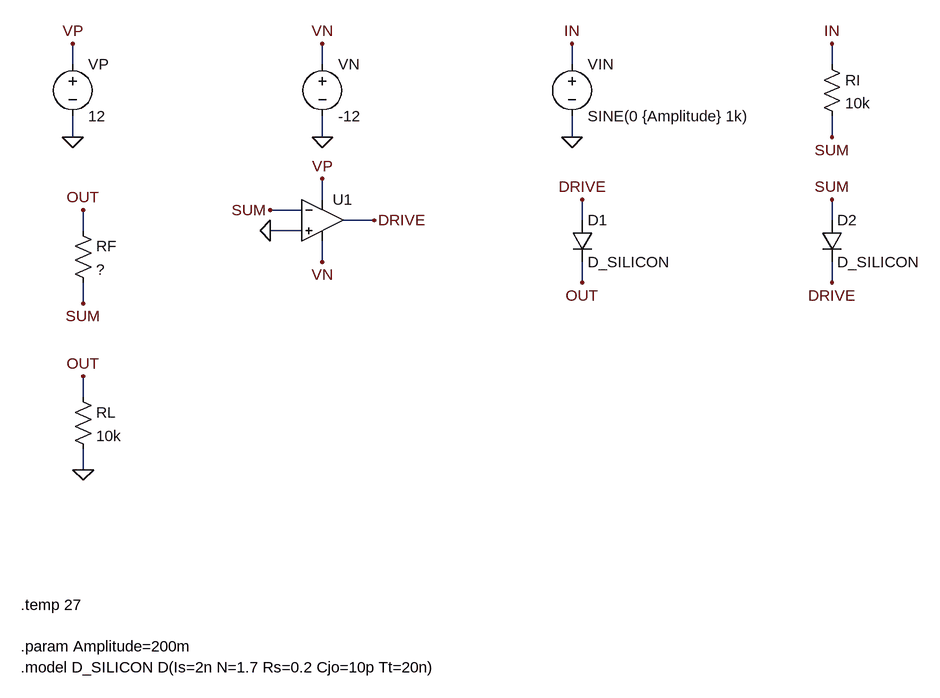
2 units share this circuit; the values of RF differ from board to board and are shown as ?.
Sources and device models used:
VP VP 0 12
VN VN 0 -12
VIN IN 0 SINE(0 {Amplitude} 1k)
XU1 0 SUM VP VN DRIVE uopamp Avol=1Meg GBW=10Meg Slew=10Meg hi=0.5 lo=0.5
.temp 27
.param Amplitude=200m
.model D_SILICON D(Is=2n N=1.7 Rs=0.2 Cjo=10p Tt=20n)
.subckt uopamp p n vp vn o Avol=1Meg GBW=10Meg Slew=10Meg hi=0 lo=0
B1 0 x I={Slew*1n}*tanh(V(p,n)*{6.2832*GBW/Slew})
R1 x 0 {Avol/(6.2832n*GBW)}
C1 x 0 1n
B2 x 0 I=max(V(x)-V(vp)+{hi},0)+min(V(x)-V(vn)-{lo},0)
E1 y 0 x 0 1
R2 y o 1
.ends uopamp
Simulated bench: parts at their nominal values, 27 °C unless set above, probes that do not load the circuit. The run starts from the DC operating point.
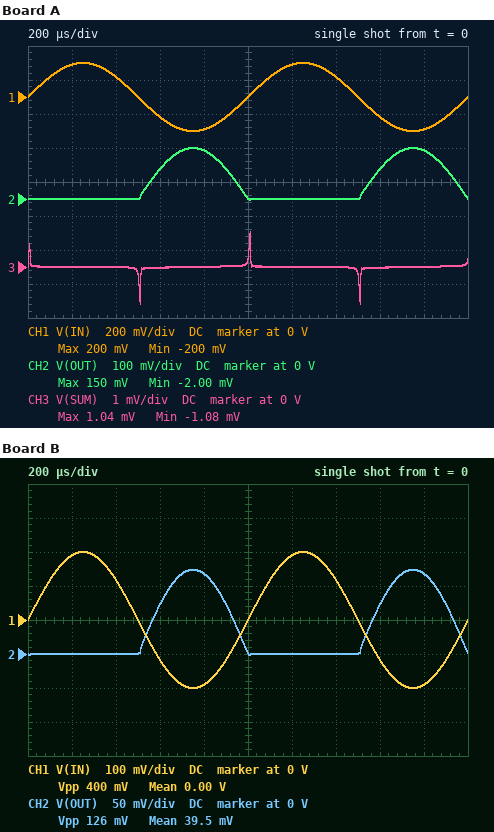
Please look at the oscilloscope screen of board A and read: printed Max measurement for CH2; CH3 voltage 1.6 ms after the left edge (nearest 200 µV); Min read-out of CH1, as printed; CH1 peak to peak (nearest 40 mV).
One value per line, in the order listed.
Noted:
150 mV
0 V
-200 mV
400 mV
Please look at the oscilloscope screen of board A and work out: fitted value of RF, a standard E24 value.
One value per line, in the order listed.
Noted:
7.5 kΩ
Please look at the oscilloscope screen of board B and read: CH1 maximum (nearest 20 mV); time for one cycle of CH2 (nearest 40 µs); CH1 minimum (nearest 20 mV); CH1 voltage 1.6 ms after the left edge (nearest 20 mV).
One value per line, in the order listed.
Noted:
200 mV
1.00 ms
-200 mV
-120 mV
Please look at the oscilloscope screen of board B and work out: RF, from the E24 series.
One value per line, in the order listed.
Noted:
6.2 kΩ
